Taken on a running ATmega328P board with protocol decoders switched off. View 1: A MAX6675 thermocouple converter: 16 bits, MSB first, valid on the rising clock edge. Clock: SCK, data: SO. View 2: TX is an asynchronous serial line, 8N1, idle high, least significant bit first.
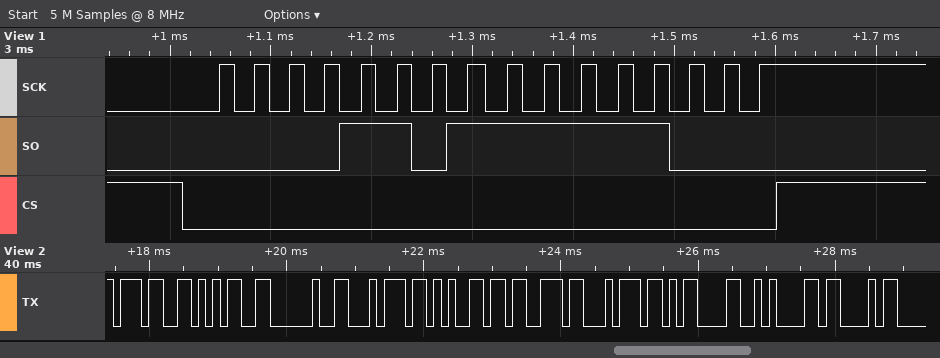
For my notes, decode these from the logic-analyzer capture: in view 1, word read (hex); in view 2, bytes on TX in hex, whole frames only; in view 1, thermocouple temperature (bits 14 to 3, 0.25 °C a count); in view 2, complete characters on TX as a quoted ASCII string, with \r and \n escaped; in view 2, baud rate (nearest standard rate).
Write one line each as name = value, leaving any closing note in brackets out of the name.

in view 1, word read = 0x0DF8
in view 2, bytes on TX in hex, whole frames only = 0x37 0x35 0x20 0x74 0x65 0x73 0x74 0x0D 0x0A 0x43
in view 1, thermocouple temperature = 111.75 °C
in view 2, complete characters on TX as a quoted ASCII string, with \r and \n escaped = "75 test\r\nC"
in view 2, baud rate = 9600 baud
